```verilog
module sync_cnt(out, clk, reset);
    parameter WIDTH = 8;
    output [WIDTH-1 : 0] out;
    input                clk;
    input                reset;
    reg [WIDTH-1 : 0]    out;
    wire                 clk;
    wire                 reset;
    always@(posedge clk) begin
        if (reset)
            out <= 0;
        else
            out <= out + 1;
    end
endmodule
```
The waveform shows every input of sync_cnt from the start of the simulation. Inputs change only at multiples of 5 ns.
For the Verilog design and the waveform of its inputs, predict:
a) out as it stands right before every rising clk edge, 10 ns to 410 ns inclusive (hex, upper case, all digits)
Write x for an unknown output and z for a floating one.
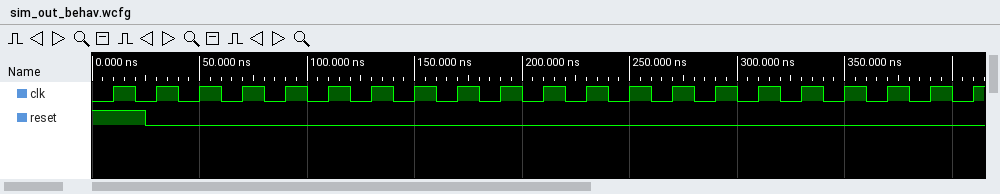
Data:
x, 00, 01, 02, 03, 04, 05, 06, 07, 08, 09, 0A, 0B, 0C, 0D, 0E, 0F, 10, 11, 12, 13
